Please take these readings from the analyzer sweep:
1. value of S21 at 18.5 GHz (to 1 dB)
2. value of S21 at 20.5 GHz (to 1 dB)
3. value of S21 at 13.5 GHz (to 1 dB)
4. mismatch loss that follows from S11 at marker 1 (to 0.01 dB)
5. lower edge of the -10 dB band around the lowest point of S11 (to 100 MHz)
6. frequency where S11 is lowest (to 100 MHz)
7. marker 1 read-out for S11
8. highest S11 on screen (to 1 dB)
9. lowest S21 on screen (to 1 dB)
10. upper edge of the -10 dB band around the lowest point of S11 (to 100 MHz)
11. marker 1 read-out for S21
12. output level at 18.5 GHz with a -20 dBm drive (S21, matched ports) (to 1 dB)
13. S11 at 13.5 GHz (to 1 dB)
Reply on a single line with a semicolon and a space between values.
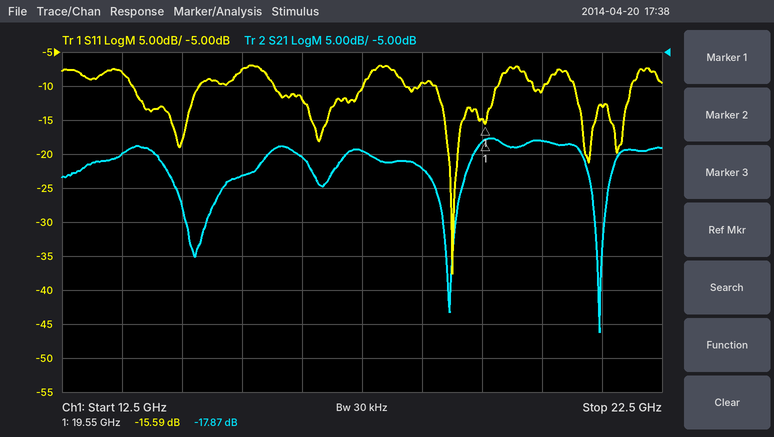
-22 dB; -18 dB; -20 dB; 0.12 dB; 18.7 GHz; 19.0 GHz; -15.59 dB; -7 dB; -46 dB; 19.8 GHz; -17.87 dB; -42 dBm; -8 dB
